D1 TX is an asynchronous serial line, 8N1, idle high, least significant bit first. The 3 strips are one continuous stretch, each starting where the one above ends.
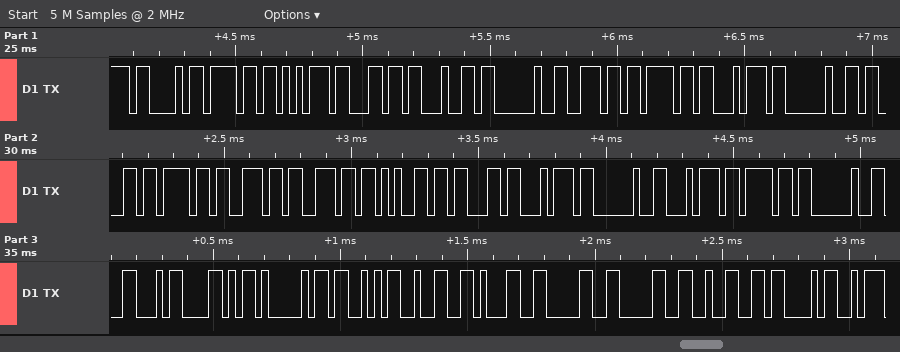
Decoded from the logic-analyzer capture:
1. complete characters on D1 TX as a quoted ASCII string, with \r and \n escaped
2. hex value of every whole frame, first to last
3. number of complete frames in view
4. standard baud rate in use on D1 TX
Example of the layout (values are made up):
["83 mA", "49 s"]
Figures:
["\"Could not connect to FXAS21002C\"", "43 6F 75 6C 64 20 6E 6F 74 20 63 6F 6E 6E 65 63 74 20 74 6F 20 46 58 41 53 32 31 30 30 32 43", "31", "38400 baud"]
